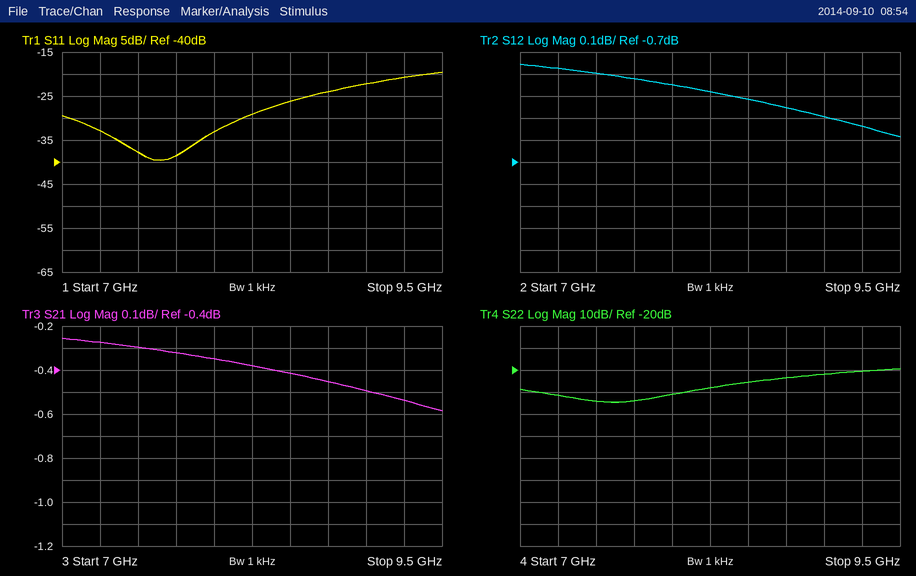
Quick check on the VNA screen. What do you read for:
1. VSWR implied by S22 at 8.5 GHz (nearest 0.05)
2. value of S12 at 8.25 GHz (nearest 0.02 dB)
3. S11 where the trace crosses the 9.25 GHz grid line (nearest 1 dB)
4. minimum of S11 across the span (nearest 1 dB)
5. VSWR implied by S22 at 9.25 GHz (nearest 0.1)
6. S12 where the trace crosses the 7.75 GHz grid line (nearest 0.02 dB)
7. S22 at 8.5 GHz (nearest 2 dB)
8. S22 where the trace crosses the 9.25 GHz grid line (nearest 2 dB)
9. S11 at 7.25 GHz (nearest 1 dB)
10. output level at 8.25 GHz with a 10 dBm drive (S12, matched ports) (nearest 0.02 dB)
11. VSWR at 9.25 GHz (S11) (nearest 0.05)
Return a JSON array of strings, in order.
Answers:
["1.10", "-0.38 dB", "-21 dB", "-40 dB", "1.2", "-0.32 dB", "-26 dB", "-20 dB", "-33 dB", "9.62 dBm", "1.20"]
